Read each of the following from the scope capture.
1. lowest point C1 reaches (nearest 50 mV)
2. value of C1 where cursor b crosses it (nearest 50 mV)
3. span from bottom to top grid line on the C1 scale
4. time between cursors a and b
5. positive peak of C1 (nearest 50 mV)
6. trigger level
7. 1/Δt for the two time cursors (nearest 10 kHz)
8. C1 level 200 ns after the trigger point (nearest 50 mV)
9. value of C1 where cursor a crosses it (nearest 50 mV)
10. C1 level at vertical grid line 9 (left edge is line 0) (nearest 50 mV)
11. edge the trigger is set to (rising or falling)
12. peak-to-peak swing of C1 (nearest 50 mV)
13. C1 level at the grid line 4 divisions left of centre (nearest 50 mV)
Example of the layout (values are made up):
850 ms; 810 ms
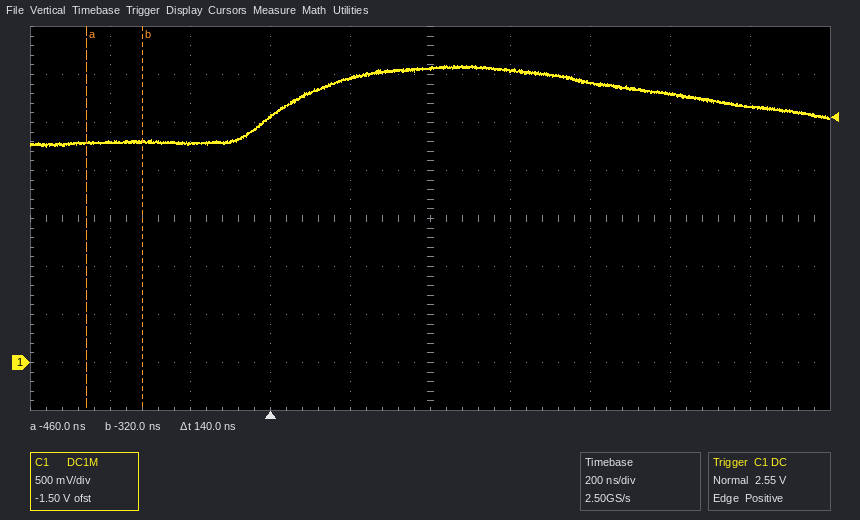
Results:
2.25 V; 2.30 V; 4 V; 140 ns; 3.10 V; 2.55 V; 7.14 MHz; 2.95 V; 2.30 V; 2.65 V; rising; 850 mV; 2.30 V
